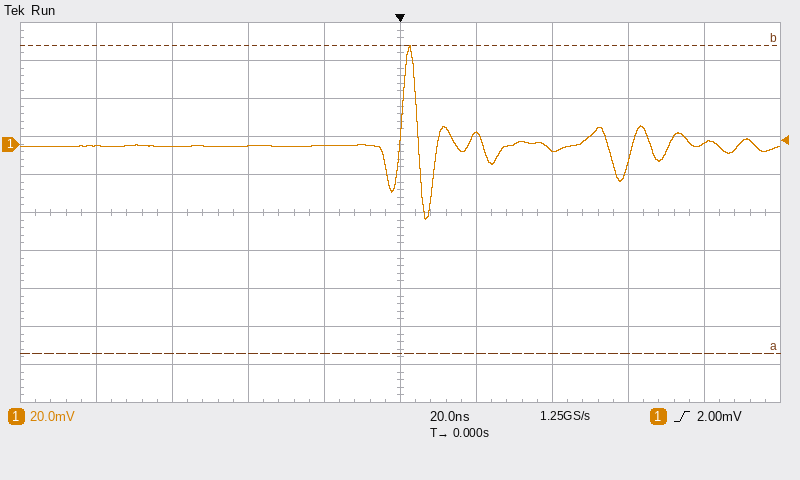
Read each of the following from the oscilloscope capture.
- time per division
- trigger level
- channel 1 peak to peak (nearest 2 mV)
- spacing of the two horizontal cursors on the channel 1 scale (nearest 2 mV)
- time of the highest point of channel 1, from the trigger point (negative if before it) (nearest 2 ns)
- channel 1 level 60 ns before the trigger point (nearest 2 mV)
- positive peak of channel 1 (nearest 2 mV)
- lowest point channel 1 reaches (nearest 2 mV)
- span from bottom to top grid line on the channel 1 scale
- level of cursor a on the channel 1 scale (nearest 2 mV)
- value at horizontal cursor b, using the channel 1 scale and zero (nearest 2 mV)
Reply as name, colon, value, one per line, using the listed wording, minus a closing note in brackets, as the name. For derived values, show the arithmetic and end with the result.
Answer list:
time per division: 20 ns
trigger level: 2.00 mV
channel 1 peak to peak: 52 mV − (-40 mV) = 92 mV
spacing of the two horizontal cursors on the channel 1 scale: 162 mV
time of the highest point of channel 1, from the trigger point (negative if before it): +2 ns
channel 1 level 60 ns before the trigger point: -2 mV
positive peak of channel 1: 52 mV
lowest point channel 1 reaches: -40 mV
span from bottom to top grid line on the channel 1 scale: 200 mV
level of cursor a on the channel 1 scale: -110 mV
value at horizontal cursor b, using the channel 1 scale and zero: 52 mV
